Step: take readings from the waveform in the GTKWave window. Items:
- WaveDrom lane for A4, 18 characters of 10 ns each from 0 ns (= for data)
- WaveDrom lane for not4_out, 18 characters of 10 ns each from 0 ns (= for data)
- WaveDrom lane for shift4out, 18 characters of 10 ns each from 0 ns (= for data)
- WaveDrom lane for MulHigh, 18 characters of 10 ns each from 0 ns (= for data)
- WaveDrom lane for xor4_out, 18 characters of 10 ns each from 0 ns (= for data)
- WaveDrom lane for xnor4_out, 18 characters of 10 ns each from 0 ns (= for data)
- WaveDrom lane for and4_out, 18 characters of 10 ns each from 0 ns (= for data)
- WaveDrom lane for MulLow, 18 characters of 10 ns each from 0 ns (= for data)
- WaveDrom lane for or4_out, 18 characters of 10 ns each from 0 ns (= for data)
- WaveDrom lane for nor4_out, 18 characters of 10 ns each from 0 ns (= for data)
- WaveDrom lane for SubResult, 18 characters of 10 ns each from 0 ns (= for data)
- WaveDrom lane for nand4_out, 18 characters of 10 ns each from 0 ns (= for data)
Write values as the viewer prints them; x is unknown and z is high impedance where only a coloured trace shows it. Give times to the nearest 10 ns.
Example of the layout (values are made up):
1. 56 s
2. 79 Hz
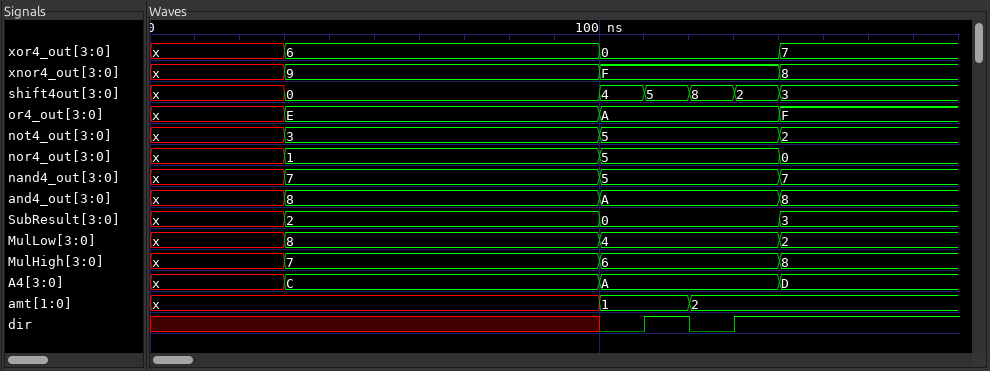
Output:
1. {name: 'A4', wave: 'x..=......=...=...', data: 'C A D'}
2. {name: 'not4_out', wave: 'x..=......=...=...', data: '3 5 2'}
3. {name: 'shift4out', wave: 'x..=......=====...', data: '0 4 5 8 2 3'}
4. {name: 'MulHigh', wave: 'x..=......=...=...', data: '7 6 8'}
5. {name: 'xor4_out', wave: 'x..=......=...=...', data: '6 0 7'}
6. {name: 'xnor4_out', wave: 'x..=......=...=...', data: '9 F 8'}
7. {name: 'and4_out', wave: 'x..=......=...=...', data: '8 A 8'}
8. {name: 'MulLow', wave: 'x..=......=...=...', data: '8 4 2'}
9. {name: 'or4_out', wave: 'x..=......=...=...', data: 'E A F'}
10. {name: 'nor4_out', wave: 'x..=......=...=...', data: '1 5 0'}
11. {name: 'SubResult', wave: 'x..=......=...=...', data: '2 0 3'}
12. {name: 'nand4_out', wave: 'x..=......=...=...', data: '7 5 7'}
